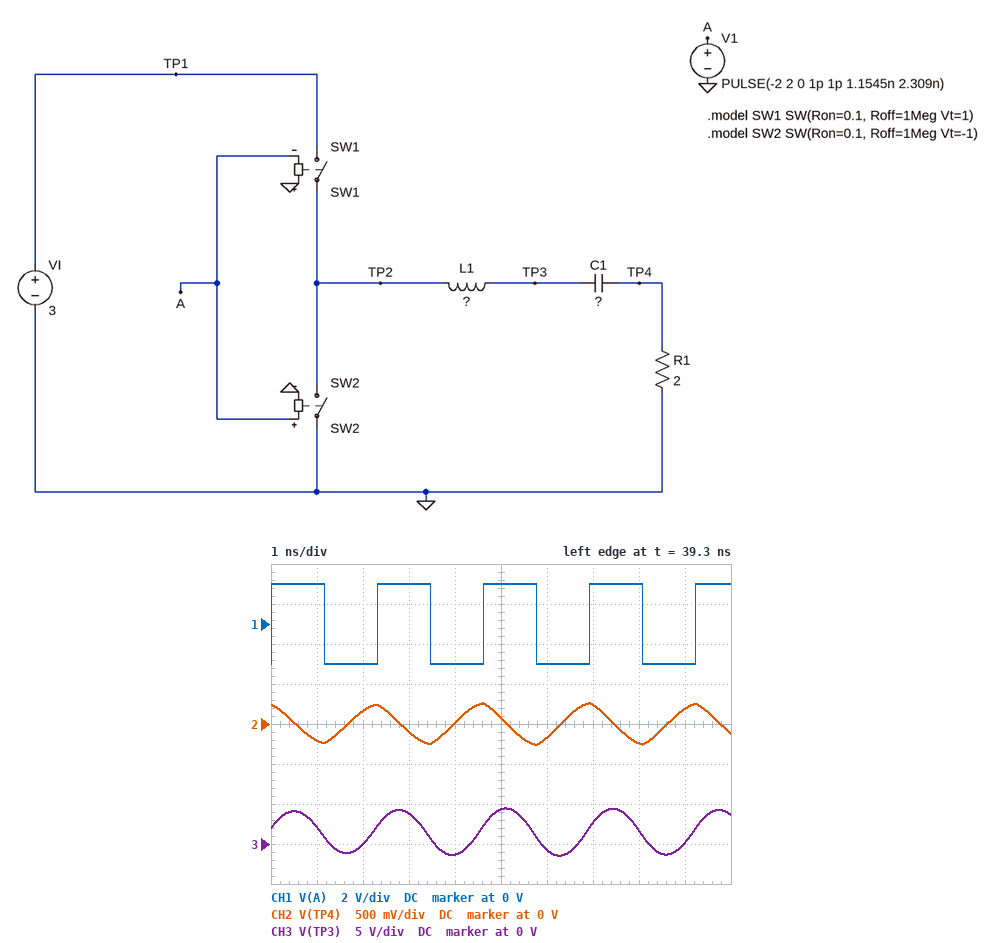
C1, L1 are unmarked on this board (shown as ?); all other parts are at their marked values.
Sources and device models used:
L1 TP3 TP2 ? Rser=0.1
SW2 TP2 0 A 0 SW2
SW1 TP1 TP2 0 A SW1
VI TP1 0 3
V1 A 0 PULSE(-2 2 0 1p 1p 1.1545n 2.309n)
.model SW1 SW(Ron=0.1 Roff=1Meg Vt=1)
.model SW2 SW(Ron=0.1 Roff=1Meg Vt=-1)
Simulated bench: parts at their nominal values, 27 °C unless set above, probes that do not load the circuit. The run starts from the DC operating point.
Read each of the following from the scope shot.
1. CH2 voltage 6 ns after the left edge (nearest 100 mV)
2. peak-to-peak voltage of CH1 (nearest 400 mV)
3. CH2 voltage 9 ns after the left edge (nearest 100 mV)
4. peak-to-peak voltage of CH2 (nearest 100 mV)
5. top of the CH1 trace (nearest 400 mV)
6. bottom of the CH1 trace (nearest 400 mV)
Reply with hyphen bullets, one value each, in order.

- -200 mV
- 4.0 V
- 200 mV
- 500 mV
- 2.0 V
- -2.0 V
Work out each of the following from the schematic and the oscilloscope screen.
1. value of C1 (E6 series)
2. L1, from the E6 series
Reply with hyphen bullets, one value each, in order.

- 15 pF
- 15 nH
